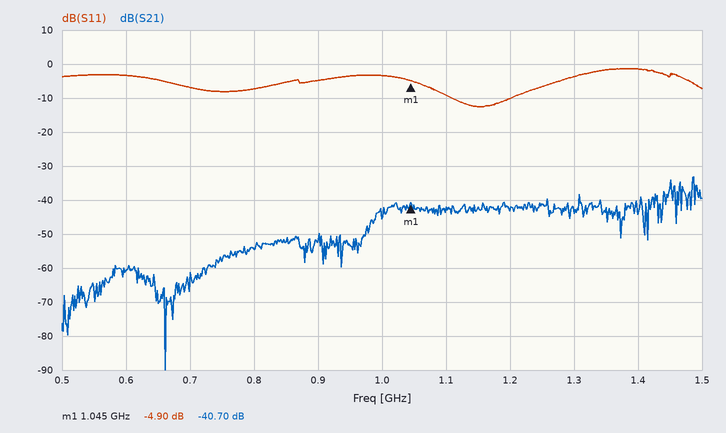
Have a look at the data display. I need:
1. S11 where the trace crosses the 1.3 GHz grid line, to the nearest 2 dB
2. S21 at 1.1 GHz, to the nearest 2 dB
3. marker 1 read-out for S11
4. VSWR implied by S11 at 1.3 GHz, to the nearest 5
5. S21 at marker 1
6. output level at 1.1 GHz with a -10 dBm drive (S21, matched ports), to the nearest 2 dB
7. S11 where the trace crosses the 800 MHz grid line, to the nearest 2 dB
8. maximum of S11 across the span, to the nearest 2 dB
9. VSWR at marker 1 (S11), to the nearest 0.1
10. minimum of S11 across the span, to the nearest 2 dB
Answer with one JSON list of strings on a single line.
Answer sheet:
["-4 dB", "-42 dB", "-4.90 dB", "5", "-40.70 dB", "-52 dBm", "-8 dB", "-2 dB", "3.6", "-12 dB"]
